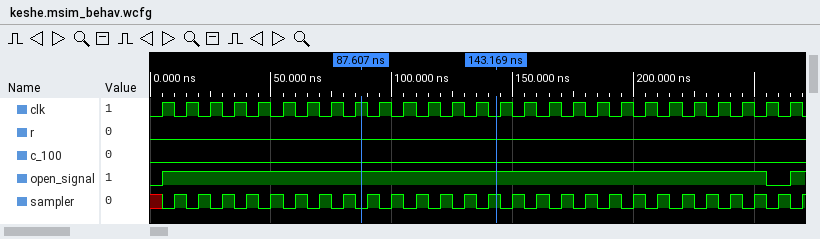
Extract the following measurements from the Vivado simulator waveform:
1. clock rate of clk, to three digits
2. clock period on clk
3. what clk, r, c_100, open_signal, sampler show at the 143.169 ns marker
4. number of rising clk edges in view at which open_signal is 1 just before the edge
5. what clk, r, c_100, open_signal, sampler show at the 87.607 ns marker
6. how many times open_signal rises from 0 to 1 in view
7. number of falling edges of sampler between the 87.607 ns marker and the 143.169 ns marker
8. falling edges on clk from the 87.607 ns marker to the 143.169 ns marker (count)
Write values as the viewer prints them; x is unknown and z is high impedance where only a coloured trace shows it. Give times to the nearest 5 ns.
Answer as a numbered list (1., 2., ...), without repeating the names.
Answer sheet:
1. 100 MHz
2. 10 ns
3. clk=0, r=0, c_100=0, open_signal=1, sampler=1
4. 25
5. clk=1, r=0, c_100=0, open_signal=1, sampler=0
6. 2
7. 5
8. 6
